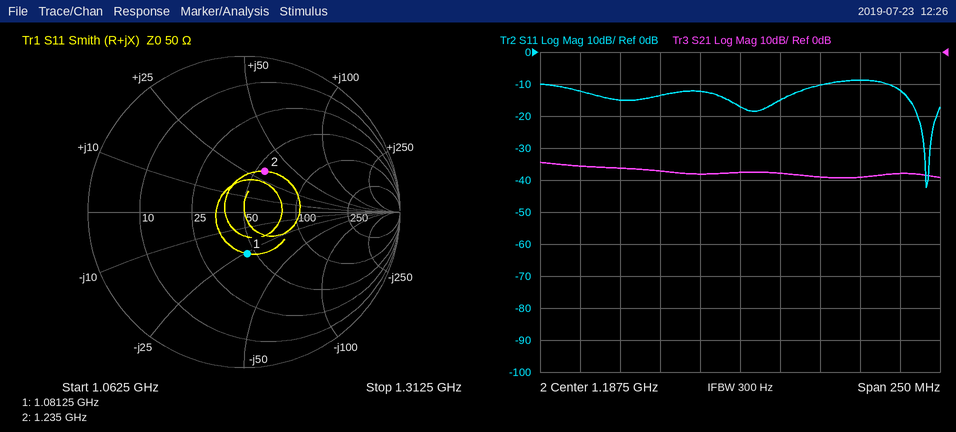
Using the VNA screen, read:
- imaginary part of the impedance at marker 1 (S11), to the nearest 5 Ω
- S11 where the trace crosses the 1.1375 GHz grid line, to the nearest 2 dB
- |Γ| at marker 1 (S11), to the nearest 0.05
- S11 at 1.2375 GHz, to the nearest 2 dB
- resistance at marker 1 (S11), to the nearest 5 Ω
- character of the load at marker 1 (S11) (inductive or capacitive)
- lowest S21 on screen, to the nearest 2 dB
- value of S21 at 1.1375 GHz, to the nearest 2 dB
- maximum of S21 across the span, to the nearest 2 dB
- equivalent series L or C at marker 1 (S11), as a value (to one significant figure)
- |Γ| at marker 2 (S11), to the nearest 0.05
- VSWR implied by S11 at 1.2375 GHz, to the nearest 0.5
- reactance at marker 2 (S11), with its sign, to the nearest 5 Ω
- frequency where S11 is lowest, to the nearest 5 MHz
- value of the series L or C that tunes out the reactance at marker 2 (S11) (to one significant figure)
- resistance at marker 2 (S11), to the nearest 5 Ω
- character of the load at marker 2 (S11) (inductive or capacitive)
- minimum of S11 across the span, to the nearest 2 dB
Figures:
-25 Ω
-14 dB
0.25
-10 dB
45 Ω
capacitive
-40 dB
-38 dB
-34 dB
6 pF
0.30
2.0
+30 Ω
1.305 GHz
4 pF
55 Ω
inductive
-42 dB
